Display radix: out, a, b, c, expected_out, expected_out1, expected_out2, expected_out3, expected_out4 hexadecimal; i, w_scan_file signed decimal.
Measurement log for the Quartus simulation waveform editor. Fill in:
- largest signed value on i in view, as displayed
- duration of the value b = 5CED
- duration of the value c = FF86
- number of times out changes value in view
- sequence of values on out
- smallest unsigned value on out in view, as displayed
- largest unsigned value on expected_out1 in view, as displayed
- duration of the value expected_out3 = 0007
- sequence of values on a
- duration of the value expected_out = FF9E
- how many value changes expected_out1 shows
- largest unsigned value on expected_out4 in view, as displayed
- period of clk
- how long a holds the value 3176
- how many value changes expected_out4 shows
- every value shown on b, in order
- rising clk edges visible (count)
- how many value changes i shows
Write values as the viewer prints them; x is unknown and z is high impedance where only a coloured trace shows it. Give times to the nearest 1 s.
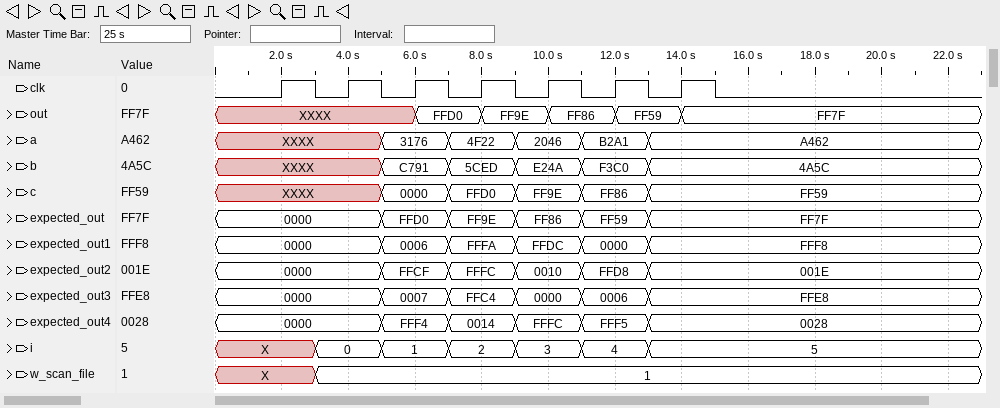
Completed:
5
2 s
2 s
5
XXXX, FFD0, FF9E, FF86, FF59, FF7F
FF59
FFFA
2 s
XXXX, 3176, 4F22, 2046, B2A1, A462
2 s
5
FFFC
2 s
2 s
5
XXXX, C791, 5CED, E24A, F3C0, 4A5C
7
6
